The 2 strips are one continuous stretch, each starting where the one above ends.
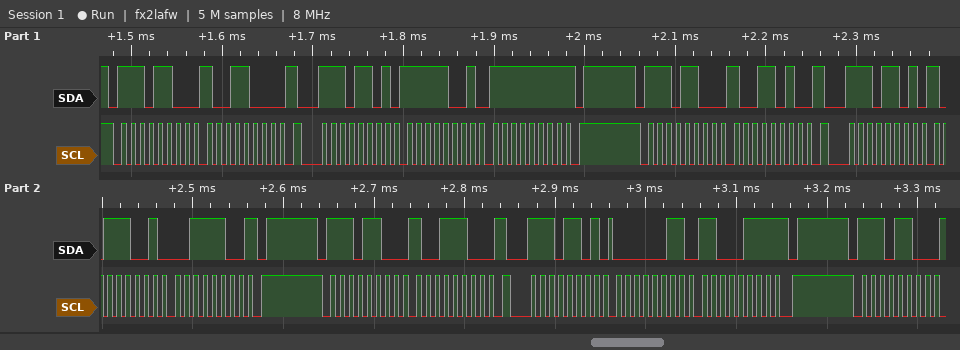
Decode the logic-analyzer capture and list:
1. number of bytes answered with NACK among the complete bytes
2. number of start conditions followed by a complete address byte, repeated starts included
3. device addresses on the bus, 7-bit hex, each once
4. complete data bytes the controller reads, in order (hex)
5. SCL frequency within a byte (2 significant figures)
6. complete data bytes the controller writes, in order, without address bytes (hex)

3
7
0x76
F9 FF B9 3C 03 C7
100 kHz
98 9A 9C
